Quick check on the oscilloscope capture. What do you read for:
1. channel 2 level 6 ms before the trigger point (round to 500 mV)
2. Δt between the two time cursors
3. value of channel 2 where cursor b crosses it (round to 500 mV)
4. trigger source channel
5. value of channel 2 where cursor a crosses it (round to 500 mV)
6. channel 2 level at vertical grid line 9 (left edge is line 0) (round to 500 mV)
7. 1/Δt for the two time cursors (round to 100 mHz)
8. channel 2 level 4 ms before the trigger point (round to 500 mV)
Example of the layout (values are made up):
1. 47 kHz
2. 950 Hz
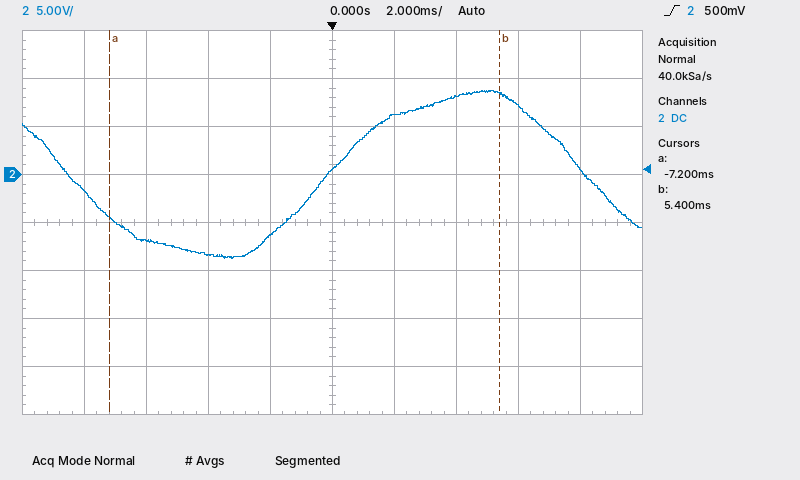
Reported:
1. -7.0 V
2. 12.6 ms
3. 8.5 V
4. channel 2
5. -4.5 V
6. 500 mV
7. 79.4 Hz
8. -8.5 V
